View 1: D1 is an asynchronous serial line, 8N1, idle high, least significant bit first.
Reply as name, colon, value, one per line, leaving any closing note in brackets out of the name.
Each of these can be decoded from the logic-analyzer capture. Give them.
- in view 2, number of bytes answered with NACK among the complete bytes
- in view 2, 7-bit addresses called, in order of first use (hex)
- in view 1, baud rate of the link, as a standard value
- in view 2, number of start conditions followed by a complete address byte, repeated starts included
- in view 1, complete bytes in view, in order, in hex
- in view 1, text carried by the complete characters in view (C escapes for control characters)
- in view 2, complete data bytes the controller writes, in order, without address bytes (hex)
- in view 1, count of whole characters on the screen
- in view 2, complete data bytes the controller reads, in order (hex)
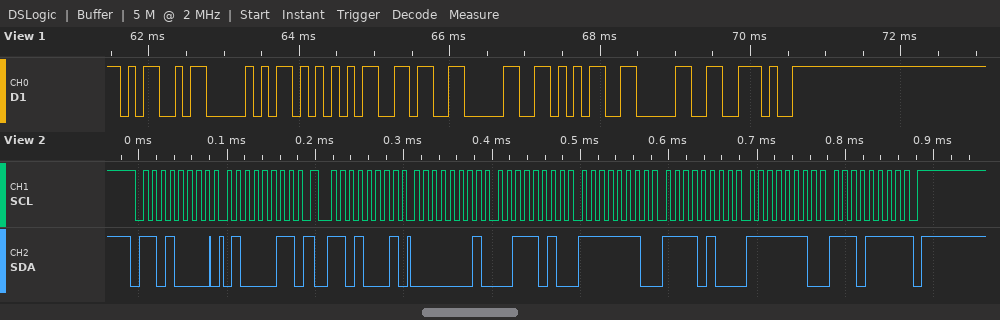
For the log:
in view 2, number of bytes answered with NACK among the complete bytes: 1
in view 2, 7-bit addresses called, in order of first use: 0x68
in view 1, baud rate of the link, as a standard value: 9600 baud
in view 2, number of start conditions followed by a complete address byte, repeated starts included: 2
in view 1, complete bytes in view, in order, in hex: 4D 50 55 36 30 35 30 2E
in view 1, text carried by the complete characters in view: "MPU6050."
in view 2, complete data bytes the controller writes, in order, without address bytes: 43
in view 1, count of whole characters on the screen: 8
in view 2, complete data bytes the controller reads, in order: 01 3A FE F4 FE EF
